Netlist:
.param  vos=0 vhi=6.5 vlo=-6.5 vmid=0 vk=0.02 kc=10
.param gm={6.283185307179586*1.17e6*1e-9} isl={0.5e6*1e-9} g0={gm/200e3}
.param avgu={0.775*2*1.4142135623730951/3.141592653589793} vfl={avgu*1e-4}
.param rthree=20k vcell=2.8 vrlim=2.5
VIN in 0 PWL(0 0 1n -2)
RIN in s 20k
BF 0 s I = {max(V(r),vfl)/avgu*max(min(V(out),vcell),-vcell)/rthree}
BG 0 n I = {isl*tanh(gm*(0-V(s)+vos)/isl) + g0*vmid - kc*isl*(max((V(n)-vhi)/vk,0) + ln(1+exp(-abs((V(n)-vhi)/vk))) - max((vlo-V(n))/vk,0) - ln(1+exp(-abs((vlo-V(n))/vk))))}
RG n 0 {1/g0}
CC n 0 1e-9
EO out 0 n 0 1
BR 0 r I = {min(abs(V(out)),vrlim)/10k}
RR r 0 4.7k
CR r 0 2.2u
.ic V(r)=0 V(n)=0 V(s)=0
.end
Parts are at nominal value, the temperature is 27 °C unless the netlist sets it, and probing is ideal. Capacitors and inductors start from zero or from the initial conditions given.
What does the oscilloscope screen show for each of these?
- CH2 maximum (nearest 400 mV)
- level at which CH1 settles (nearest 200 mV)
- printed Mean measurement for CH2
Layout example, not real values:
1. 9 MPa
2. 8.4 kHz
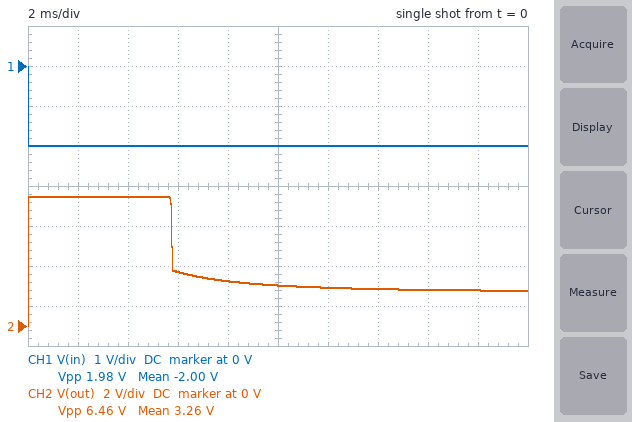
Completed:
1. 6.4 V
2. -2.0 V
3. 3.26 V
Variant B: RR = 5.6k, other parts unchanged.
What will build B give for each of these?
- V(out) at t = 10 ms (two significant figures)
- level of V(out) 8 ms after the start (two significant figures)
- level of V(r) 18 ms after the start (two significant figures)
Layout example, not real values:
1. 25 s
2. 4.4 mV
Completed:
1. 1.9 V
2. 2.1 V
3. 840 mV
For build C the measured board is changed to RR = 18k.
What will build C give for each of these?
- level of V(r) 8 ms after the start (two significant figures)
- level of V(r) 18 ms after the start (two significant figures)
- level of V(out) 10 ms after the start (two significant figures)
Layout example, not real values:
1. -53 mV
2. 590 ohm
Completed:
1. 770 mV
2. 1.2 V
3. 1.6 V
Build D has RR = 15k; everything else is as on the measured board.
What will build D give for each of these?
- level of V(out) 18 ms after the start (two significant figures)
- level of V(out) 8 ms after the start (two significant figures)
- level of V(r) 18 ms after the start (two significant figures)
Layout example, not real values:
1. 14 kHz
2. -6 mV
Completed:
1. 1.2 V
2. 1.8 V
3. 1.1 V
